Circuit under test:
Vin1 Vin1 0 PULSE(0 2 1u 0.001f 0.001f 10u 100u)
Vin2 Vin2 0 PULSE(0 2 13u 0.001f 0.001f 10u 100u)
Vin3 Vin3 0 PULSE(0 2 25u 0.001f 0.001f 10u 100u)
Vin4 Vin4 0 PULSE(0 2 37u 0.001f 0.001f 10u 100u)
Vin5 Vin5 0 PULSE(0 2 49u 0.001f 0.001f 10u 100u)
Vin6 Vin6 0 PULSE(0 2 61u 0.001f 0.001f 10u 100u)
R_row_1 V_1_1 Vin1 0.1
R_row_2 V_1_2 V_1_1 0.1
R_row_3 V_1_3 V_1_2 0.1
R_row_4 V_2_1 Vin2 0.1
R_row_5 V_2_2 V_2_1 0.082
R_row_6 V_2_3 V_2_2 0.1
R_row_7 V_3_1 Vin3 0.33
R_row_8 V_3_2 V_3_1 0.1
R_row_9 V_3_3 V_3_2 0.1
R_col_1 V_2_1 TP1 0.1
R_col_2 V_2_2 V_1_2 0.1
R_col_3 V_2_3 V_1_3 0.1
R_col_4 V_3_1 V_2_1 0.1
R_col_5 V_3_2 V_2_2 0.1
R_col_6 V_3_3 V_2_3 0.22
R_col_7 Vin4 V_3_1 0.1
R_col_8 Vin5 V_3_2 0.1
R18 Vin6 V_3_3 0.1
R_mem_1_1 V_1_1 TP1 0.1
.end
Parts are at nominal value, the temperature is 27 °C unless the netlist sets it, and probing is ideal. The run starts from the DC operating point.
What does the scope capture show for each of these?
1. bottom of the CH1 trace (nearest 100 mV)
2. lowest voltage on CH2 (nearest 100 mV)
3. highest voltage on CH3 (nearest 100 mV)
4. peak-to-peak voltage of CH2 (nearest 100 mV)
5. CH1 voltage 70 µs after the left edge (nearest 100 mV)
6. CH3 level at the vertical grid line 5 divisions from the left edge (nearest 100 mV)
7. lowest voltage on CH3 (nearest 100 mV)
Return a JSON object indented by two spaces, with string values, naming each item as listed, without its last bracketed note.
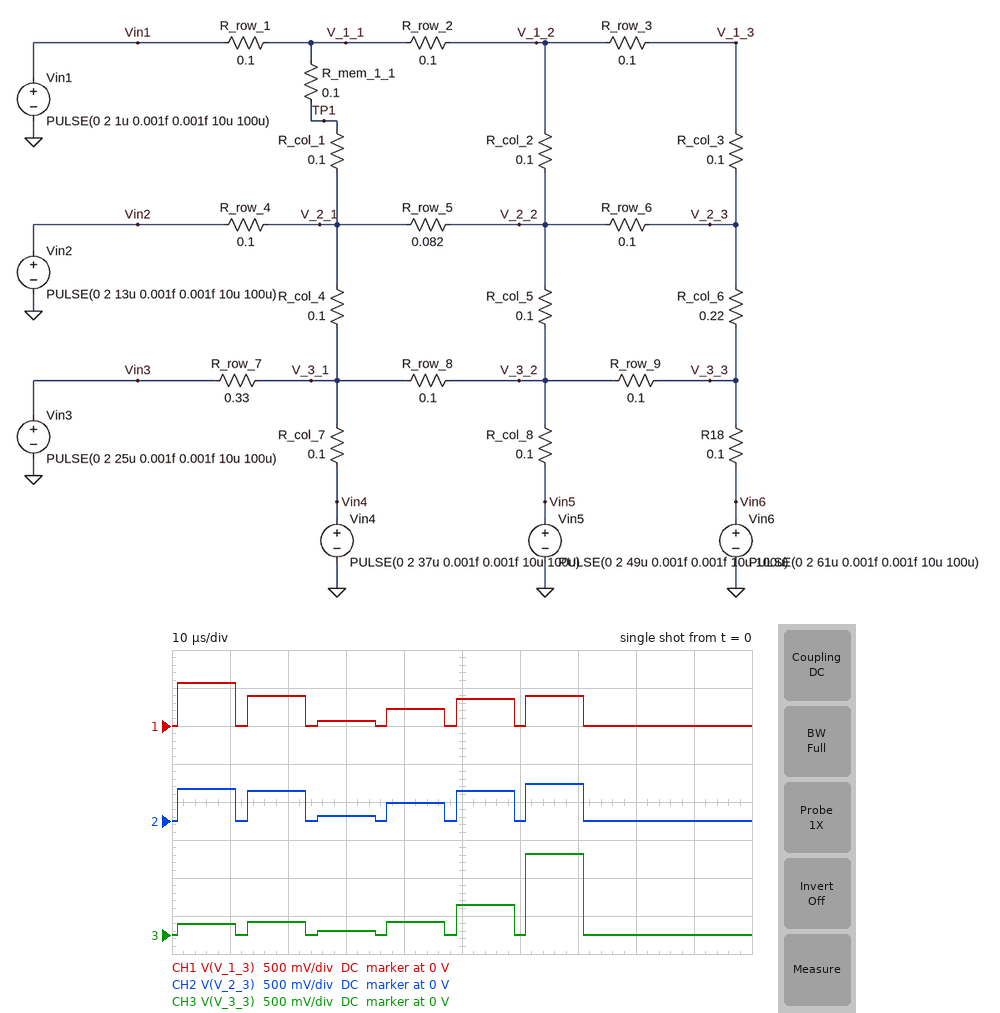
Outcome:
{
  "bottom of the CH1 trace": "0 V",
  "lowest voltage on CH2": "0 V",
  "highest voltage on CH3": "1.1 V",
  "peak-to-peak voltage of CH2": "500 mV",
  "CH1 voltage 70 µs after the left edge": "400 mV",
  "CH3 level at the vertical grid line 5 divisions from the left edge": "400 mV",
  "lowest voltage on CH3": "0 V"
}
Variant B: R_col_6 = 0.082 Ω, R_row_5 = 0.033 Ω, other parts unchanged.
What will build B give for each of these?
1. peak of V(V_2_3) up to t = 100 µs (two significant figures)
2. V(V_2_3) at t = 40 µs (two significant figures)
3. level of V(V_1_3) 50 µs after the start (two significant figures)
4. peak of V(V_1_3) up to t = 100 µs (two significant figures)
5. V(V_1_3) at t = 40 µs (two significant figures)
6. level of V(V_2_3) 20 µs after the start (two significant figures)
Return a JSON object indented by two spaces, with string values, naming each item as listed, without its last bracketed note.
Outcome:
{
  "peak of V(V_2_3) up to t = 100 µs": "620 mV",
  "V(V_2_3) at t = 40 µs": "230 mV",
  "level of V(V_1_3) 50 µs after the start": "320 mV",
  "peak of V(V_1_3) up to t = 100 µs": "500 mV",
  "V(V_1_3) at t = 40 µs": "220 mV",
  "level of V(V_2_3) 20 µs after the start": "390 mV"
}
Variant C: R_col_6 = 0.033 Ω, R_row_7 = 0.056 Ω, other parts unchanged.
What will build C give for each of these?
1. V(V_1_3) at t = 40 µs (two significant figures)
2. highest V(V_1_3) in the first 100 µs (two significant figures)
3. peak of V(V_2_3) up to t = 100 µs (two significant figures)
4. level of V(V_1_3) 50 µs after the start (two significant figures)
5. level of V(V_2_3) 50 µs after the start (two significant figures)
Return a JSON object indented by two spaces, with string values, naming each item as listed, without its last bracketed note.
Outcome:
{
  "V(V_1_3) at t = 40 µs": "130 mV",
  "highest V(V_1_3) in the first 100 µs": "570 mV",
  "peak of V(V_2_3) up to t = 100 µs": "750 mV",
  "level of V(V_1_3) 50 µs after the start": "320 mV",
  "level of V(V_2_3) 50 µs after the start": "360 mV"
}
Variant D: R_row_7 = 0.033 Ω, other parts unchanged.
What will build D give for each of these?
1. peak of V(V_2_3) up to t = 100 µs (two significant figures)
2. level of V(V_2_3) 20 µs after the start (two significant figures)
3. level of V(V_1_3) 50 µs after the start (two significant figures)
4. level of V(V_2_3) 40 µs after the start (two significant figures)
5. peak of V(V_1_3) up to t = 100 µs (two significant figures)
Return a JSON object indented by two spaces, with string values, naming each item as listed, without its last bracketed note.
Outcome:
{
  "peak of V(V_2_3) up to t = 100 µs": "460 mV",
  "level of V(V_2_3) 20 µs after the start": "340 mV",
  "level of V(V_1_3) 50 µs after the start": "310 mV",
  "level of V(V_2_3) 40 µs after the start": "110 mV",
  "peak of V(V_1_3) up to t = 100 µs": "540 mV"
}
